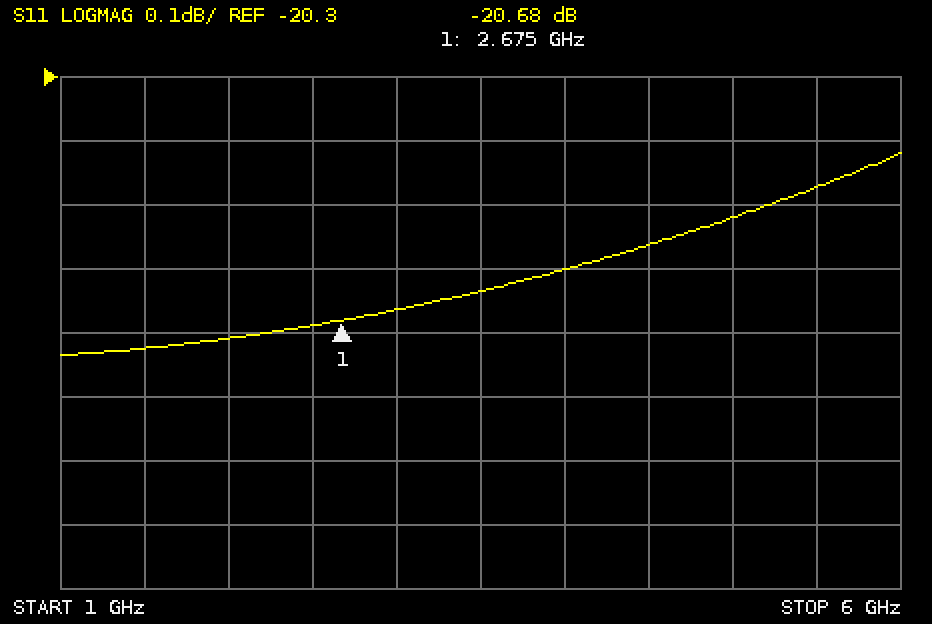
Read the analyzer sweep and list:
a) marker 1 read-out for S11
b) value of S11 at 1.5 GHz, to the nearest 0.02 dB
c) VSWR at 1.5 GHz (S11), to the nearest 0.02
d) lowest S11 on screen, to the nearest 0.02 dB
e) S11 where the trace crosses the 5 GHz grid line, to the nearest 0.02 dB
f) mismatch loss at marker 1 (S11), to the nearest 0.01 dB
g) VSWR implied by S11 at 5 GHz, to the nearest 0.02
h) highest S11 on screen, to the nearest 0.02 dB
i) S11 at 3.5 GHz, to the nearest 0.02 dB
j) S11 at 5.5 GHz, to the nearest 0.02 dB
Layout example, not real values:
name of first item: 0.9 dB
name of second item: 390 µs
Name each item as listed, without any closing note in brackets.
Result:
marker 1 read-out for S11: -20.68 dB
value of S11 at 1.5 GHz, to the nearest 0.02 dB: -20.72 dB
VSWR at 1.5 GHz (S11), to the nearest 0.02: 1.20
lowest S11 on screen, to the nearest 0.02 dB: -20.74 dB
S11 where the trace crosses the 5 GHz grid line, to the nearest 0.02 dB: -20.52 dB
mismatch loss at marker 1 (S11), to the nearest 0.01 dB: 0.04 dB
VSWR implied by S11 at 5 GHz, to the nearest 0.02: 1.20
highest S11 on screen, to the nearest 0.02 dB: -20.42 dB
S11 at 3.5 GHz, to the nearest 0.02 dB: -20.64 dB
S11 at 5.5 GHz, to the nearest 0.02 dB: -20.48 dB
